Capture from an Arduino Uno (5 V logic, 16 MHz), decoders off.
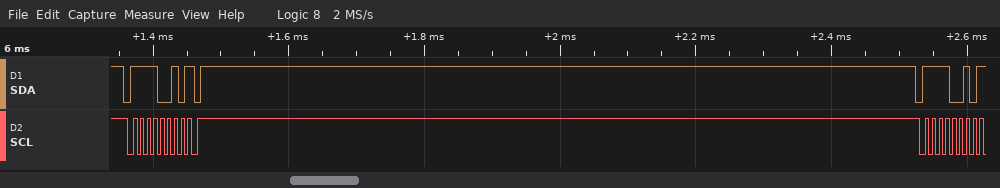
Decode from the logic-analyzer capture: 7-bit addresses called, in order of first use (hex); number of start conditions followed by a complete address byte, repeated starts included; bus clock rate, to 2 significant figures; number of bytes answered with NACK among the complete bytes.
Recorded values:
0x79
2
100 kHz
2
